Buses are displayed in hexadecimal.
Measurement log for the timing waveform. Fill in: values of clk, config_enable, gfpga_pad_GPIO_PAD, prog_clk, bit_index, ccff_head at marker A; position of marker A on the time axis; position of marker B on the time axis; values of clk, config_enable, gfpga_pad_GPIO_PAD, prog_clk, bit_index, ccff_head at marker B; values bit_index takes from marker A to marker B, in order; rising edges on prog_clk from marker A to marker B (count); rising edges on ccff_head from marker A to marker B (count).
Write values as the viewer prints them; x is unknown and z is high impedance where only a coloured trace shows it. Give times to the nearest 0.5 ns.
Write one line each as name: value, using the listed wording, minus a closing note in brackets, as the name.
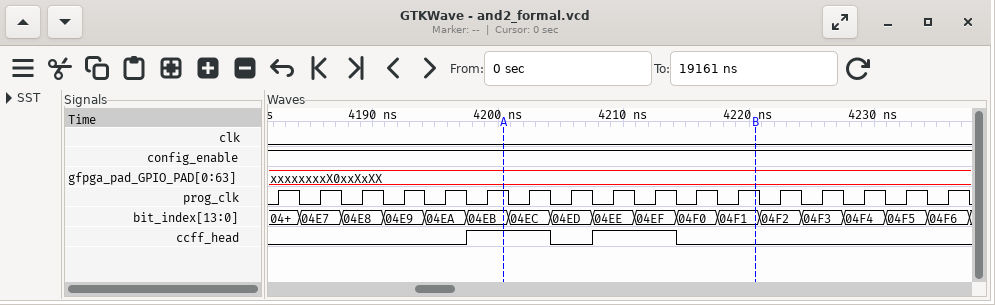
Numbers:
values of clk, config_enable, gfpga_pad_GPIO_PAD, prog_clk, bit_index, ccff_head at marker A: clk=0, config_enable=1, gfpga_pad_GPIO_PAD=xxxxxxxxX0xxXxXX, prog_clk=1, bit_index=04EB, ccff_head=1
position of marker A on the time axis: 4200.5 ns
position of marker B on the time axis: 4220.5 ns
values of clk, config_enable, gfpga_pad_GPIO_PAD, prog_clk, bit_index, ccff_head at marker B: clk=0, config_enable=1, gfpga_pad_GPIO_PAD=xxxxxxxxX0xxXxXX, prog_clk=1, bit_index=04F1, ccff_head=0
values bit_index takes from marker A to marker B, in order: 04EB, 04EC, 04ED, 04EE, 04EF, 04F0, 04F1
rising edges on prog_clk from marker A to marker B: 6
rising edges on ccff_head from marker A to marker B: 1
